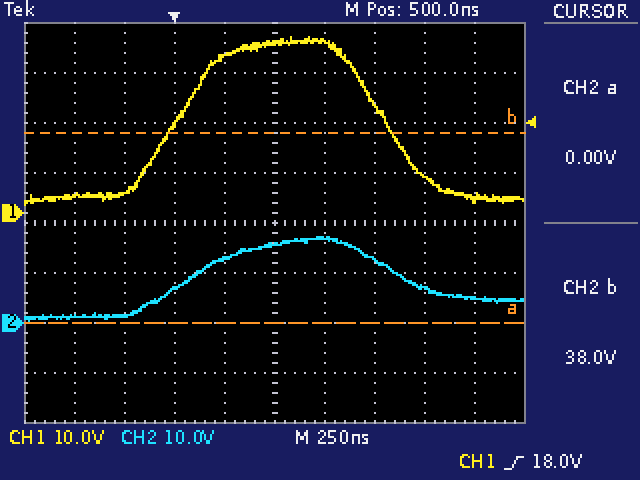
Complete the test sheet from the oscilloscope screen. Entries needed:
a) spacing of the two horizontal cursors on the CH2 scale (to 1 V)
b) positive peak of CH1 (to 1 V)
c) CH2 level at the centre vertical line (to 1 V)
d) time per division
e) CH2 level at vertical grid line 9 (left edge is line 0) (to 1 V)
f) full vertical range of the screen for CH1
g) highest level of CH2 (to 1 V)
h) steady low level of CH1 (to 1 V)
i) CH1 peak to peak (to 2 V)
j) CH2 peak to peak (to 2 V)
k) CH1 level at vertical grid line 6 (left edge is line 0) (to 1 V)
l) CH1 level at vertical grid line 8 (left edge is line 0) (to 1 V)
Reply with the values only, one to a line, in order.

38 V
35 V
16 V
250 ns
5 V
80 V
17 V
3 V
34 V
16 V
34 V
7 V
